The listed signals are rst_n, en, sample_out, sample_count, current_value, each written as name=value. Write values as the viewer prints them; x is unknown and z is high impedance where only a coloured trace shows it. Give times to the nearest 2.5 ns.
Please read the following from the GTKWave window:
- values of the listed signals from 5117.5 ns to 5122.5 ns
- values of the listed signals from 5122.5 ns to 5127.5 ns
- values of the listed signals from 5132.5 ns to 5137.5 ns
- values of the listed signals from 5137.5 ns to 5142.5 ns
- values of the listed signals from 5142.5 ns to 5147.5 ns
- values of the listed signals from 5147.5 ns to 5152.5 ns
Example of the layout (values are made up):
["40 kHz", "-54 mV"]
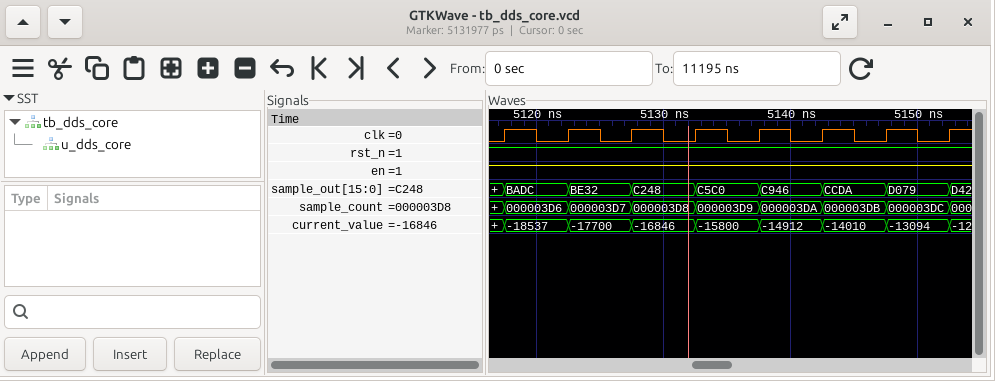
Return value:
["rst_n=1, en=1, sample_out=BADC, sample_count=000003D6, current_value=-18537", "rst_n=1, en=1, sample_out=BE32, sample_count=000003D7, current_value=-17700", "rst_n=1, en=1, sample_out=C5C0, sample_count=000003D9, current_value=-15800", "rst_n=1, en=1, sample_out=C946, sample_count=000003DA, current_value=-14912", "rst_n=1, en=1, sample_out=CCDA, sample_count=000003DB, current_value=-14010", "rst_n=1, en=1, sample_out=D079, sample_count=000003DC, current_value=-13094"]
